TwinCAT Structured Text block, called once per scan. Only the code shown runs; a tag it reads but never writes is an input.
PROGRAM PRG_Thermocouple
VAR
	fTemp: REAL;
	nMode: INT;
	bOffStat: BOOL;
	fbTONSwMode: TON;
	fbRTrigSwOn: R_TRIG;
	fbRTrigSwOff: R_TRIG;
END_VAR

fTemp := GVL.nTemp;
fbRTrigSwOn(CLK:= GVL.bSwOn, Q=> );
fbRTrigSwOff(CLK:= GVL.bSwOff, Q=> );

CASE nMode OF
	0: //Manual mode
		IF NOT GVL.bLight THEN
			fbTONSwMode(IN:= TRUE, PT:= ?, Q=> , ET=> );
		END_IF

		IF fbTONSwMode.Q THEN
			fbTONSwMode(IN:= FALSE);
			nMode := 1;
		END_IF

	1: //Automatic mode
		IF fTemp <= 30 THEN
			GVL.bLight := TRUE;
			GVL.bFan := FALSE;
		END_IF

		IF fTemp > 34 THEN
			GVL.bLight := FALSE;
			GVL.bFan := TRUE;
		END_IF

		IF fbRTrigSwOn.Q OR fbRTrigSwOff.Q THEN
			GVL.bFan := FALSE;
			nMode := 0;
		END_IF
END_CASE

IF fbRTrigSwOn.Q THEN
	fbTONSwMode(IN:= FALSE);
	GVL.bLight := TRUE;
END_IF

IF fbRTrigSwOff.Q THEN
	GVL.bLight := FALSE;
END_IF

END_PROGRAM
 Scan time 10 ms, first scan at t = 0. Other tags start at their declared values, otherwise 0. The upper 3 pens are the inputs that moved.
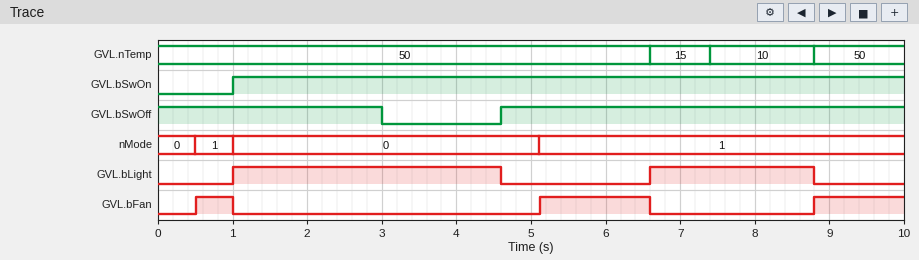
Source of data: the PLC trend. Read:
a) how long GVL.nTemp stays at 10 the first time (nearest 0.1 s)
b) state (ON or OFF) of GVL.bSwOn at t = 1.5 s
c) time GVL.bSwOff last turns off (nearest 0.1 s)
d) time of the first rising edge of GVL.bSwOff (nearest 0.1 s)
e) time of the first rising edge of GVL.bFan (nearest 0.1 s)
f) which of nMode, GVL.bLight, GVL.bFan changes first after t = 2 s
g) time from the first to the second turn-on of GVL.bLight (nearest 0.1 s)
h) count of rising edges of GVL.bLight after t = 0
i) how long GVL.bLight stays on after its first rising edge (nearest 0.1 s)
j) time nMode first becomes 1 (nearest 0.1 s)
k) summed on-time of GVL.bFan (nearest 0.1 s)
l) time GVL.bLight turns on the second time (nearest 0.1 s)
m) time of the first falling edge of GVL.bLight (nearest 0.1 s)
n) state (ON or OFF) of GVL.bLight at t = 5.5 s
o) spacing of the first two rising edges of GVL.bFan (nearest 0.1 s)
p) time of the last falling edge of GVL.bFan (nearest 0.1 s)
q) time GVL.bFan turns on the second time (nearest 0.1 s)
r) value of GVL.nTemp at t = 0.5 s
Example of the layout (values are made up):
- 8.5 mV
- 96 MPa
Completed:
- 1.4 s
- ON
- 3.0 s
- 4.6 s
- 0.5 s
- GVL.bLight
- 5.6 s
- 2
- 3.6 s
- 0.5 s
- 3.2 s
- 6.6 s
- 4.6 s
- OFF
- 4.6 s
- 6.6 s
- 5.1 s
- 50
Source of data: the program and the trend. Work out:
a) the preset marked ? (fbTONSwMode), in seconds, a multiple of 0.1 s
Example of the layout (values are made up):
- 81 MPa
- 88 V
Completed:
- 0.5 s
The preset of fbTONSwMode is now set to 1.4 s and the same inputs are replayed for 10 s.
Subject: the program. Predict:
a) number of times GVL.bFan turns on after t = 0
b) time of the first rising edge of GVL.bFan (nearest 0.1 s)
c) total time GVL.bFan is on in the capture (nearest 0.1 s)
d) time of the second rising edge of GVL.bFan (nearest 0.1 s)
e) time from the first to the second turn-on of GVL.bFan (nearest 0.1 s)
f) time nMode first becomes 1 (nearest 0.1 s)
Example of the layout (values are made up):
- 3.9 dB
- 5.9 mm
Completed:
- 2
- 6.0 s
- 1.8 s
- 8.8 s
- 2.8 s
- 6.0 s
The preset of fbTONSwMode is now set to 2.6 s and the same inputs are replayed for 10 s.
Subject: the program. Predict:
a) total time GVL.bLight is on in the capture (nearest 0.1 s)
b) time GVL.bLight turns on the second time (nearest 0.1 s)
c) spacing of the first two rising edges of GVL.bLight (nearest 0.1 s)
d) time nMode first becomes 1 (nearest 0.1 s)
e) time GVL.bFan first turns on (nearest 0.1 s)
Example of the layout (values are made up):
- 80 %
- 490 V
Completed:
- 5.2 s
- 7.2 s
- 6.2 s
- 7.2 s
- 8.8 s
